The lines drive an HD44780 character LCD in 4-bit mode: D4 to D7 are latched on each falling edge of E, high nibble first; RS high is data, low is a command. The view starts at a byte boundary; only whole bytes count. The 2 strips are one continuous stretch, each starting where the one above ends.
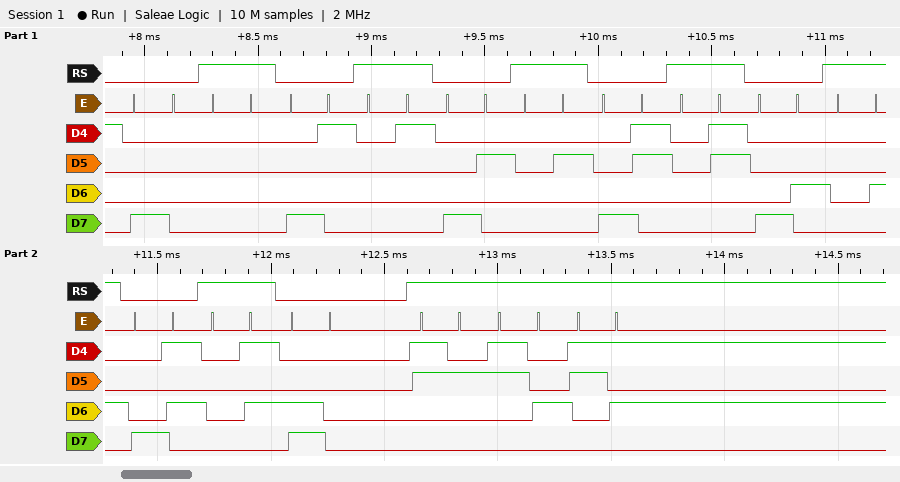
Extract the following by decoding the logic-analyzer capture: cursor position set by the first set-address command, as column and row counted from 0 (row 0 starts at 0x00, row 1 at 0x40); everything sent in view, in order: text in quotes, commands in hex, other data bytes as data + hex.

column 0, row 0
0x80 data 00 0x81 data 01 0x82 data 02 0x83 data 03 0x84 data 04 0x85 data 05 0xC0 "245"
